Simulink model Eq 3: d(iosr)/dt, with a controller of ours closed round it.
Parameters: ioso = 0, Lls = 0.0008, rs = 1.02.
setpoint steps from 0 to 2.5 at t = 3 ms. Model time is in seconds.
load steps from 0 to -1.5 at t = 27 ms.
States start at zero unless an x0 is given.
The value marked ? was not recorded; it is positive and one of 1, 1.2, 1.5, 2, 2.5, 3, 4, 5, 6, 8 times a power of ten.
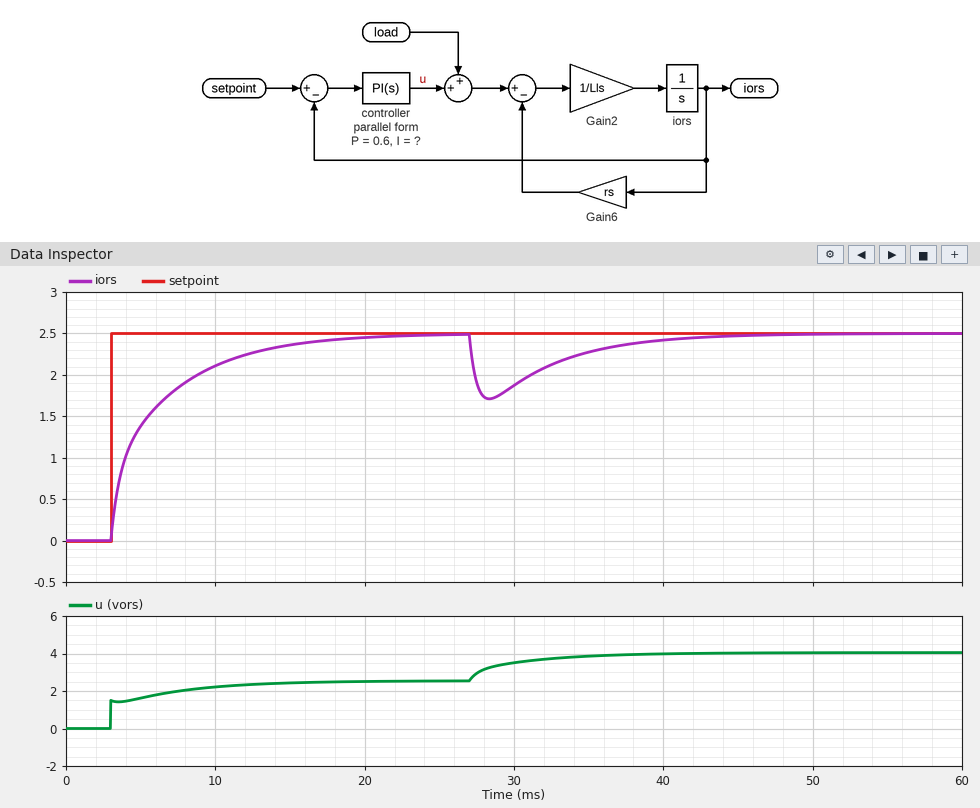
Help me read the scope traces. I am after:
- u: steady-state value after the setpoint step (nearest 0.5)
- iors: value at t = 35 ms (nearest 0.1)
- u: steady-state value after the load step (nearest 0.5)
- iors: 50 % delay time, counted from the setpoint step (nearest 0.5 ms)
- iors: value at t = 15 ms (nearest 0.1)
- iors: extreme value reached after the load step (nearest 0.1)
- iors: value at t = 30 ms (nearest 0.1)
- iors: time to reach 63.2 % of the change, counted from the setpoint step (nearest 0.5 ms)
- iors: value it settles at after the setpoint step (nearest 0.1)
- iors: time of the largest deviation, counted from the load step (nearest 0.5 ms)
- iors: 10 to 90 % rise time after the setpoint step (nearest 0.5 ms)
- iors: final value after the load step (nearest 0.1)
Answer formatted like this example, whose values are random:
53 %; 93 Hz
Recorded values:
2.5; 2.3; 4.0; 1.5 ms; 2.4; 1.7; 1.9; 3.0 ms; 2.5; 1.5 ms; 9.0 ms; 2.5
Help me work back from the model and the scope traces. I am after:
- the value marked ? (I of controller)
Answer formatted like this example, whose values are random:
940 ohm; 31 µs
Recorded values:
300
